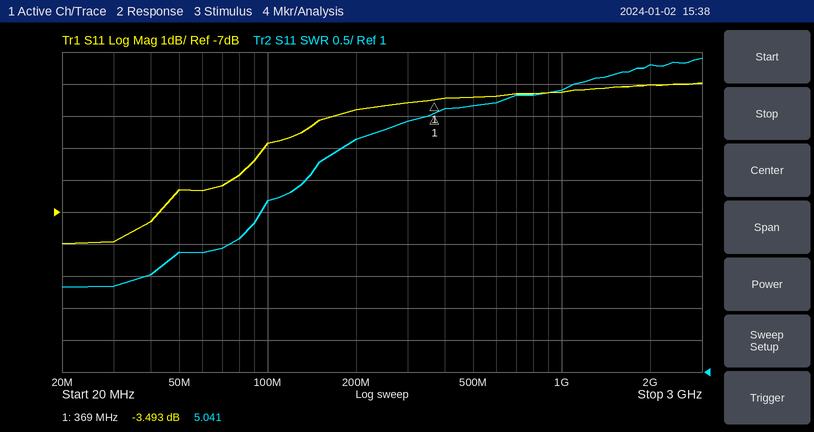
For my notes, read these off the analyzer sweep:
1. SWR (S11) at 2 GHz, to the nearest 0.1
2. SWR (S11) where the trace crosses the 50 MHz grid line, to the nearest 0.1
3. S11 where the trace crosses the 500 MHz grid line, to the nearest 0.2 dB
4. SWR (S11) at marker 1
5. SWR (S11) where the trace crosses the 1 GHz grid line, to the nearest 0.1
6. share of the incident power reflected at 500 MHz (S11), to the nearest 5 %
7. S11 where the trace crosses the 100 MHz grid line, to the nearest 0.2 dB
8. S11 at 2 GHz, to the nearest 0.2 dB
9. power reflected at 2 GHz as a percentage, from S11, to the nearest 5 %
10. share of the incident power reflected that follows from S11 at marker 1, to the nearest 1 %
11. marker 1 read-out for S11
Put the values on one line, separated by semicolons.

5.8; 2.9; -3.4 dB; 5.041; 5.4; 45 %; -4.8 dB; -3.0 dB; 50 %; 45 %; -3.493 dB
